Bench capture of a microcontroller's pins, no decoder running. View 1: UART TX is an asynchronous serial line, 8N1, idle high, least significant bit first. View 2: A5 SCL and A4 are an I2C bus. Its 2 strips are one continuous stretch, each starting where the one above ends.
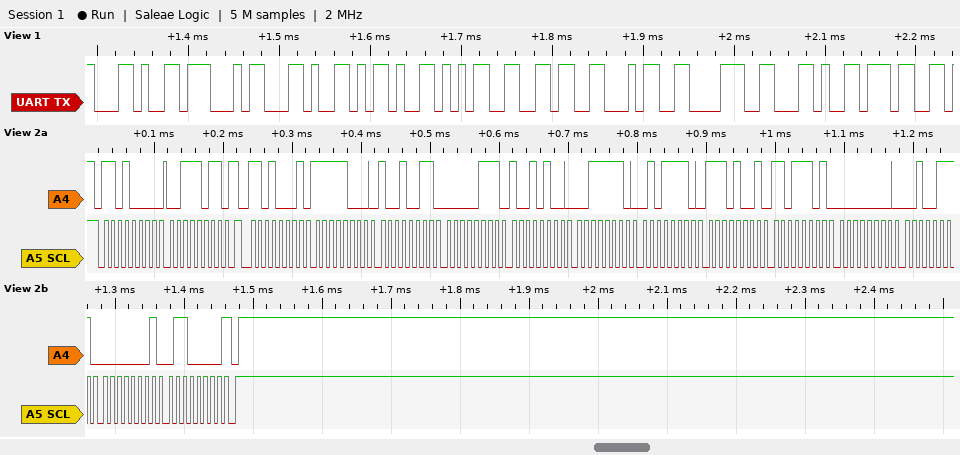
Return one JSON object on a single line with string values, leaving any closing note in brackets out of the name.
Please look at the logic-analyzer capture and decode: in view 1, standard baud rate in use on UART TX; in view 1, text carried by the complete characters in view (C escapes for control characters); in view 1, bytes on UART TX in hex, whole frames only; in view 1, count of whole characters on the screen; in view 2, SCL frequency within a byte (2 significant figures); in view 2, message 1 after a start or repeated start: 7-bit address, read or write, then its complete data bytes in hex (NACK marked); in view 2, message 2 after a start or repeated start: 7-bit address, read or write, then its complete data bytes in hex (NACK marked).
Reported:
{"in view 1, standard baud rate in use on UART TX": "115200 baud", "in view 1, text carried by the complete characters in view": "\",G,-5648,7\"", "in view 1, bytes on UART TX in hex, whole frames only": "2C 47 2C 2D 35 36 34 38 2C 37", "in view 1, count of whole characters on the screen": "10", "in view 2, SCL frequency within a byte": "100 kHz", "in view 2, message 1 after a start or repeated start: 7-bit address, read or write, then its complete data bytes in hex": "0x68 write: 3B", "in view 2, message 2 after a start or repeated start: 7-bit address, read or write, then its complete data bytes in hex": "0x68 read: F8 93 07 94 3E 5E E9 DD 00 27 01 60 NACK"}
